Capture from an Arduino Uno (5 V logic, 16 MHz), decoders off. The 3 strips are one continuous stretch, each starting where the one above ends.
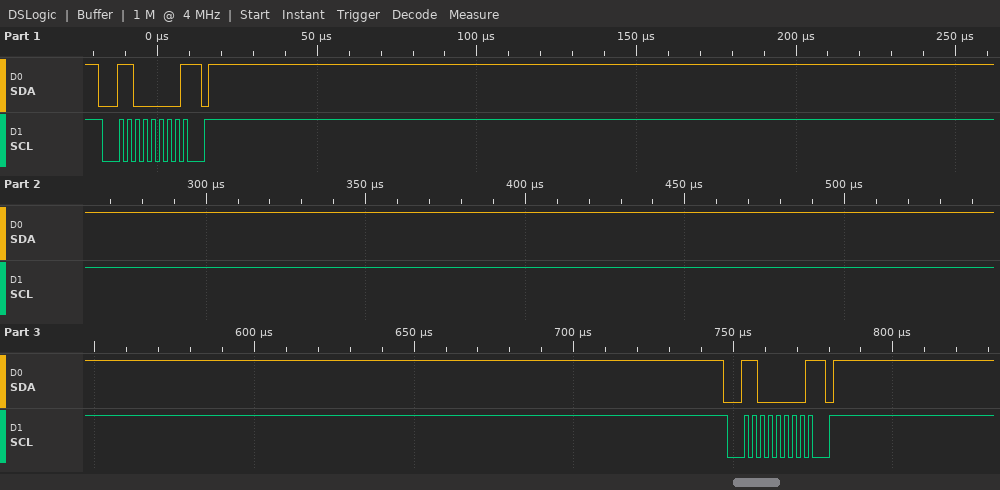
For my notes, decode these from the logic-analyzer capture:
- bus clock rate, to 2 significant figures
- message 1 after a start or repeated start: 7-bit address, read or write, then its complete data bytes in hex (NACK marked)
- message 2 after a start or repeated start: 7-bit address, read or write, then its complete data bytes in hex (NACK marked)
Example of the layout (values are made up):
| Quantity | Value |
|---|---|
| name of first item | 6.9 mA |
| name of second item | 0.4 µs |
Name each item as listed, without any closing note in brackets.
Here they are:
| Quantity | Value |
|---|---|
| bus clock rate, to 2 significant figures | 400 kHz |
| message 1 after a start or repeated start: 7-bit address, read or write, then its complete data bytes in hex | 0x60 write NACK |
| message 2 after a start or repeated start: 7-bit address, read or write, then its complete data bytes in hex | 0x60 write NACK |
